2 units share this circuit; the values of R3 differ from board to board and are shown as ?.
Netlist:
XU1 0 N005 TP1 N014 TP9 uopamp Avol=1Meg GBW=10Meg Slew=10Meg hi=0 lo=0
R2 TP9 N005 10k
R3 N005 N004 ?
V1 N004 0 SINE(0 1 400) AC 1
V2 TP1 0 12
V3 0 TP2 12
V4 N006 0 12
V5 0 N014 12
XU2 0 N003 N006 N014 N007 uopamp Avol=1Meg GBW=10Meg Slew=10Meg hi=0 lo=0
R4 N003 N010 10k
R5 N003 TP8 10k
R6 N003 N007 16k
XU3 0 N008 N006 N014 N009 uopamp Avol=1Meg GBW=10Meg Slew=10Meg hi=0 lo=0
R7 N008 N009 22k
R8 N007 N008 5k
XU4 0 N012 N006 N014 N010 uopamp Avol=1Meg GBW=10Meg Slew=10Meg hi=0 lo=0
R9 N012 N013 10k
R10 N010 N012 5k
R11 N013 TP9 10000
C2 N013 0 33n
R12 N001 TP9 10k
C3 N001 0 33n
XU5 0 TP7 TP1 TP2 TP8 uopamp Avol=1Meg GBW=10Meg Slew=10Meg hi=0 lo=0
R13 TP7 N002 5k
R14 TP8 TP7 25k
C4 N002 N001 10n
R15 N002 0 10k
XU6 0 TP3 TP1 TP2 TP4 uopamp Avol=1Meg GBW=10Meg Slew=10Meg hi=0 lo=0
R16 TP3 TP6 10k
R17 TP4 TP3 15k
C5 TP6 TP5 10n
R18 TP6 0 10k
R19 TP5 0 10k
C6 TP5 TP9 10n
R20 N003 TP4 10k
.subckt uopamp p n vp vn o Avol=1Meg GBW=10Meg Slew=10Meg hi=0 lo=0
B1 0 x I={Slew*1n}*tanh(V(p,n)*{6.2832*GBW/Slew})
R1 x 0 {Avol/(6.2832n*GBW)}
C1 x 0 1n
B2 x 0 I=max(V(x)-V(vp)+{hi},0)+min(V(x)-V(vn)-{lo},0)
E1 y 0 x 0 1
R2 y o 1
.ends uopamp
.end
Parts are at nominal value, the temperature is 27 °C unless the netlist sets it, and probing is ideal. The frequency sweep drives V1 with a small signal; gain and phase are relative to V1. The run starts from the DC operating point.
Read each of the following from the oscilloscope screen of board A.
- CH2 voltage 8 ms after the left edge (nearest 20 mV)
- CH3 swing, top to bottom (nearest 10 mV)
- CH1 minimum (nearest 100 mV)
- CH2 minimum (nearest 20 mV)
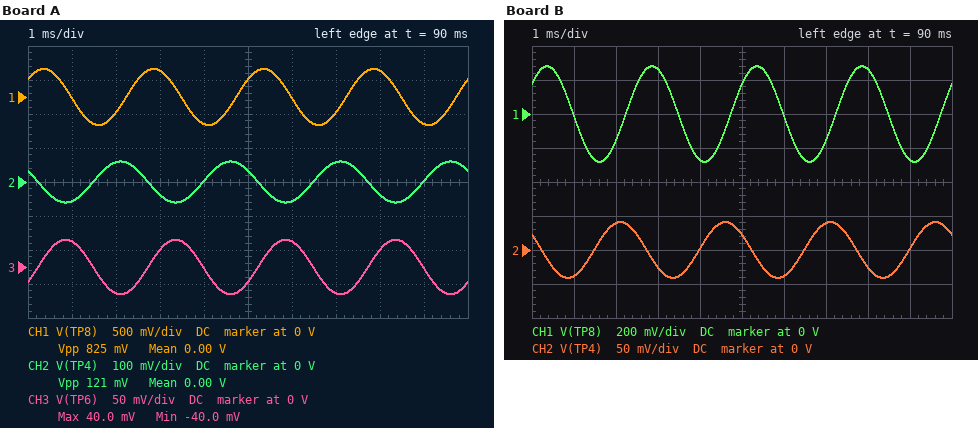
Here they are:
-40 mV
80 mV
-400 mV
-60 mV
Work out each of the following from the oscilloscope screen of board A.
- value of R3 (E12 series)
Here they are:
6.8 kΩ
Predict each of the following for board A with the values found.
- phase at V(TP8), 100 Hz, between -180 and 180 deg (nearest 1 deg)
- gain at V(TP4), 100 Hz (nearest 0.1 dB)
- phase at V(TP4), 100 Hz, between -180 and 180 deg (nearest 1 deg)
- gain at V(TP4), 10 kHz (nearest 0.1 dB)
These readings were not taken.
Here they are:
74 deg
-47.3 dB
171 deg
5.0 dB
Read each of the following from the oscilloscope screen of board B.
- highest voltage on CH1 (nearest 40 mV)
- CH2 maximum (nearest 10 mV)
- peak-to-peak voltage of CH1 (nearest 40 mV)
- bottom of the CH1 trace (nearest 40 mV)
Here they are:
280 mV
40 mV
560 mV
-280 mV
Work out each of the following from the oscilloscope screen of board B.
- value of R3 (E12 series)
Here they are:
10 kΩ
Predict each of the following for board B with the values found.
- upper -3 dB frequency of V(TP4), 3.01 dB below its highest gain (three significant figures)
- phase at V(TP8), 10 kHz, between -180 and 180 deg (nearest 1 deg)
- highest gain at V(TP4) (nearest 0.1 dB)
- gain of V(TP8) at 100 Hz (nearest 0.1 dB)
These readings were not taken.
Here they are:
2.86 MHz
-56 deg
3.5 dB
-19.9 dB
